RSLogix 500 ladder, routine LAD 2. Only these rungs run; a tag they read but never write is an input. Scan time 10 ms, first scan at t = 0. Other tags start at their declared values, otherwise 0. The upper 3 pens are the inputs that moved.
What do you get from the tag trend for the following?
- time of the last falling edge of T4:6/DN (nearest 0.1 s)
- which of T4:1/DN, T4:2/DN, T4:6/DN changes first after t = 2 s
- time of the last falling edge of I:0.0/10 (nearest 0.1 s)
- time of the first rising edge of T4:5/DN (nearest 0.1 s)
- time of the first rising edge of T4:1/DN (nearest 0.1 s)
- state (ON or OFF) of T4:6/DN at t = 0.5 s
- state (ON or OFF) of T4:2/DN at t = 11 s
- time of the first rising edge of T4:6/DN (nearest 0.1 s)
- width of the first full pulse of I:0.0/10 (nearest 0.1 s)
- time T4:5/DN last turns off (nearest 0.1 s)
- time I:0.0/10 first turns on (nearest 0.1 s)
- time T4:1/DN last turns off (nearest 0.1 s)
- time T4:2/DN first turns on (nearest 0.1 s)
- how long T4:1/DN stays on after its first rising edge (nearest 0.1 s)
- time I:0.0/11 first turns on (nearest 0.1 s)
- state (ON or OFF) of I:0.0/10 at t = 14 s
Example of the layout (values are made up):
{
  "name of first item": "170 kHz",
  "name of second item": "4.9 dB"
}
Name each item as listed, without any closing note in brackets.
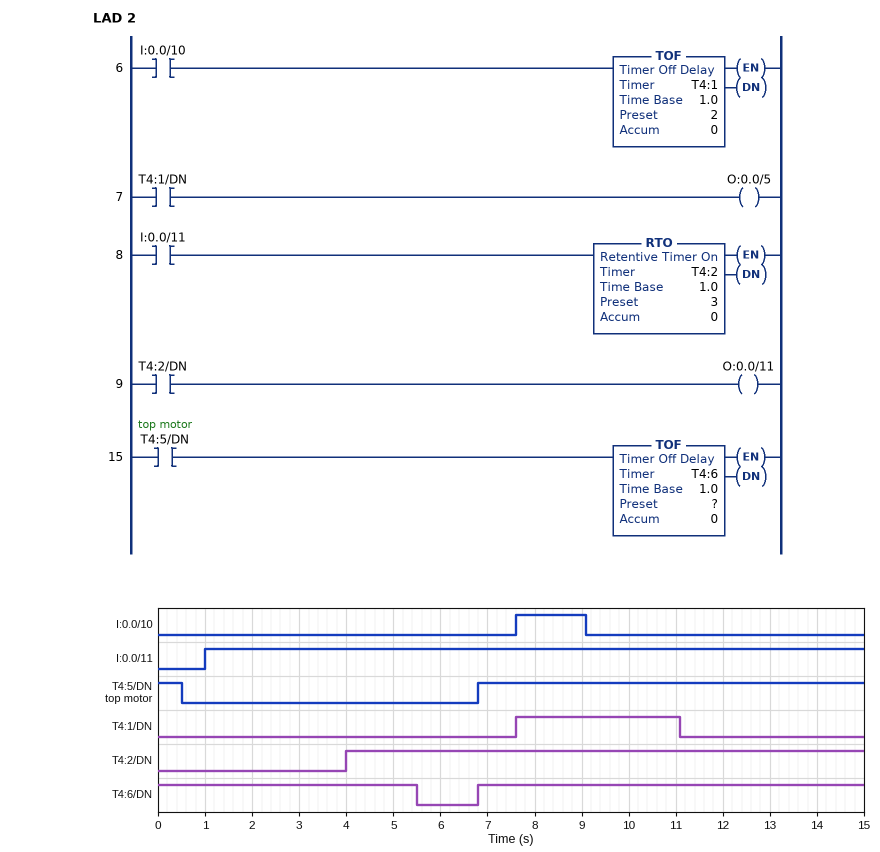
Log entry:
{
  "time of the last falling edge of T4:6/DN": "5.5 s",
  "which of T4:1/DN, T4:2/DN, T4:6/DN changes first after t = 2 s": "T4:2/DN",
  "time of the last falling edge of I:0.0/10": "9.1 s",
  "time of the first rising edge of T4:5/DN": "6.8 s",
  "time of the first rising edge of T4:1/DN": "7.6 s",
  "state (ON or OFF) of T4:6/DN at t = 0.5 s": "ON",
  "state (ON or OFF) of T4:2/DN at t = 11 s": "ON",
  "time of the first rising edge of T4:6/DN": "6.8 s",
  "width of the first full pulse of I:0.0/10": "1.5 s",
  "time T4:5/DN last turns off": "0.5 s",
  "time I:0.0/10 first turns on": "7.6 s",
  "time T4:1/DN last turns off": "11.1 s",
  "time T4:2/DN first turns on": "4.0 s",
  "how long T4:1/DN stays on after its first rising edge": "3.5 s",
  "time I:0.0/11 first turns on": "1.0 s",
  "state (ON or OFF) of I:0.0/10 at t = 14 s": "OFF"
}
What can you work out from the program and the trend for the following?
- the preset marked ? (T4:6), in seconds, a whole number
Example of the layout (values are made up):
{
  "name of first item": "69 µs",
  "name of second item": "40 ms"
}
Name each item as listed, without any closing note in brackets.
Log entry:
{
  "the preset marked ? (T4:6), in seconds, a whole number": "5 s"
}
